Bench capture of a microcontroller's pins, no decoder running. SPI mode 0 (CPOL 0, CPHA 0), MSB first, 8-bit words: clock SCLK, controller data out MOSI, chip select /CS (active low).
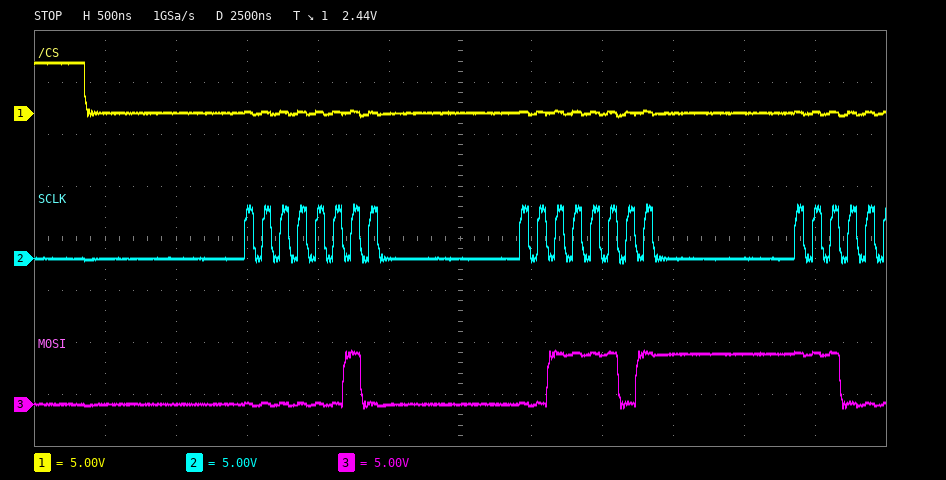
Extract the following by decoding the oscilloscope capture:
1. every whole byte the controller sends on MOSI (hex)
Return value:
0x02 0x3D
